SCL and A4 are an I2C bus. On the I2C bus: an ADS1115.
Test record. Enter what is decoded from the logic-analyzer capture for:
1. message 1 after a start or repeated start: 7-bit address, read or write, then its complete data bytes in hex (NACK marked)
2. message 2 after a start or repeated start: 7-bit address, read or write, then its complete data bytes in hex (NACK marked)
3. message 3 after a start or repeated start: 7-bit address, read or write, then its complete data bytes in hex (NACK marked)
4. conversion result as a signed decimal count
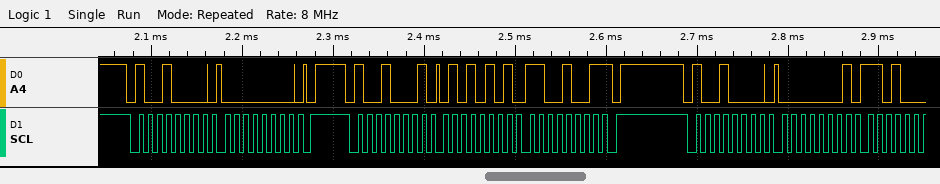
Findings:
0x48 write: 00
0x48 read: 55 C9 NACK
0x48 write: 01
21961
